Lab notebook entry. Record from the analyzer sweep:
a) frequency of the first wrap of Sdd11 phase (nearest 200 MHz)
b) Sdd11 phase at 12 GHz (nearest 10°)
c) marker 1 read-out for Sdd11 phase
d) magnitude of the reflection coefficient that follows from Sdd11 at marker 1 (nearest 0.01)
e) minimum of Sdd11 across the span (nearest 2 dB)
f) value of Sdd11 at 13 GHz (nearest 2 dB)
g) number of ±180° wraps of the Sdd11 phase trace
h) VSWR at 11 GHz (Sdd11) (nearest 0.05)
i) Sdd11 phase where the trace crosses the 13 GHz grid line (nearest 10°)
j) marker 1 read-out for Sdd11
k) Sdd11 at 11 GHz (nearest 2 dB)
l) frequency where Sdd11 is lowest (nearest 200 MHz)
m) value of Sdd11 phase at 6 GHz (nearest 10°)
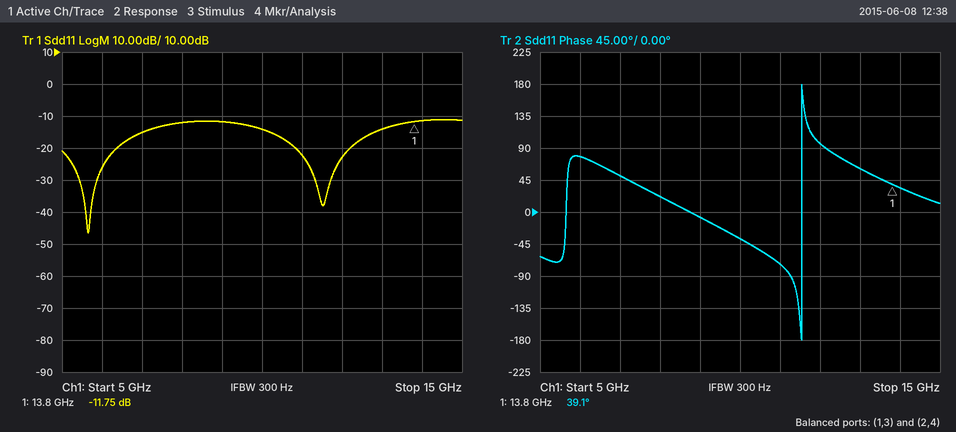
11.6 GHz
100°
39.1°
0.26
-46 dB
-14 dB
1
1.15
60°
-11.75 dB
-22 dB
5.6 GHz
80°
